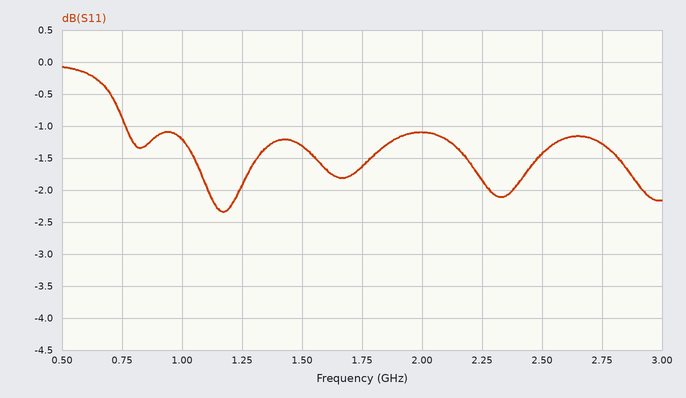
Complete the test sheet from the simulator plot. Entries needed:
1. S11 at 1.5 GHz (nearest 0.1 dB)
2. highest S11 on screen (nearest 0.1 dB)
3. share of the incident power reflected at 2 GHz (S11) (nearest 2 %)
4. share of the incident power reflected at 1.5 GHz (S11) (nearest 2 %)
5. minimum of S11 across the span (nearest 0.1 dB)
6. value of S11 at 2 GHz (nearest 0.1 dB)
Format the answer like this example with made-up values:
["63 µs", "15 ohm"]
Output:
["-1.3 dB", "-0.1 dB", "78 %", "74 %", "-2.3 dB", "-1.1 dB"]
